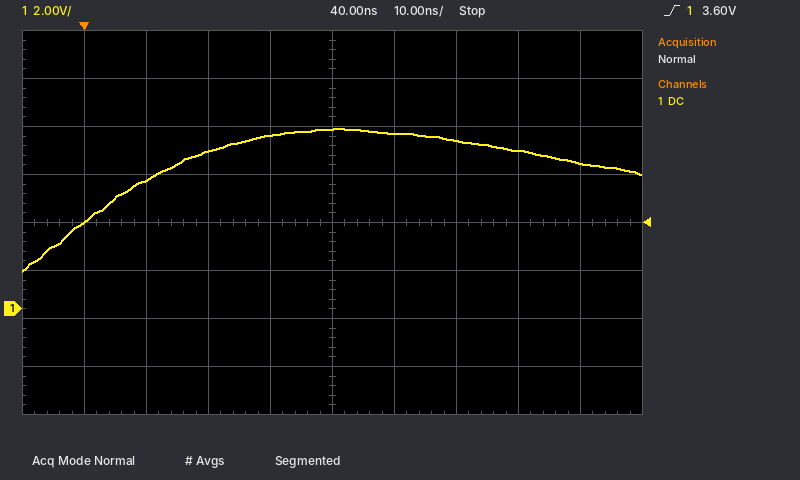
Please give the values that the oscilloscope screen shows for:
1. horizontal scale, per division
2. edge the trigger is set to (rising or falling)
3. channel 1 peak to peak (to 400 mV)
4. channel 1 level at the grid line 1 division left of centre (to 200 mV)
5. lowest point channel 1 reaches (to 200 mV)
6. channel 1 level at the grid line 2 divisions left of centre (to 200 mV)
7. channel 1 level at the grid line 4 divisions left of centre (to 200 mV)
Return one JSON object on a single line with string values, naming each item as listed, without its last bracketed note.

{"horizontal scale, per division": "10 ns", "edge the trigger is set to": "rising", "channel 1 peak to peak": "6.0 V", "channel 1 level at the grid line 1 division left of centre": "7.2 V", "lowest point channel 1 reaches": "1.6 V", "channel 1 level at the grid line 2 divisions left of centre": "6.6 V", "channel 1 level at the grid line 4 divisions left of centre": "3.6 V"}
